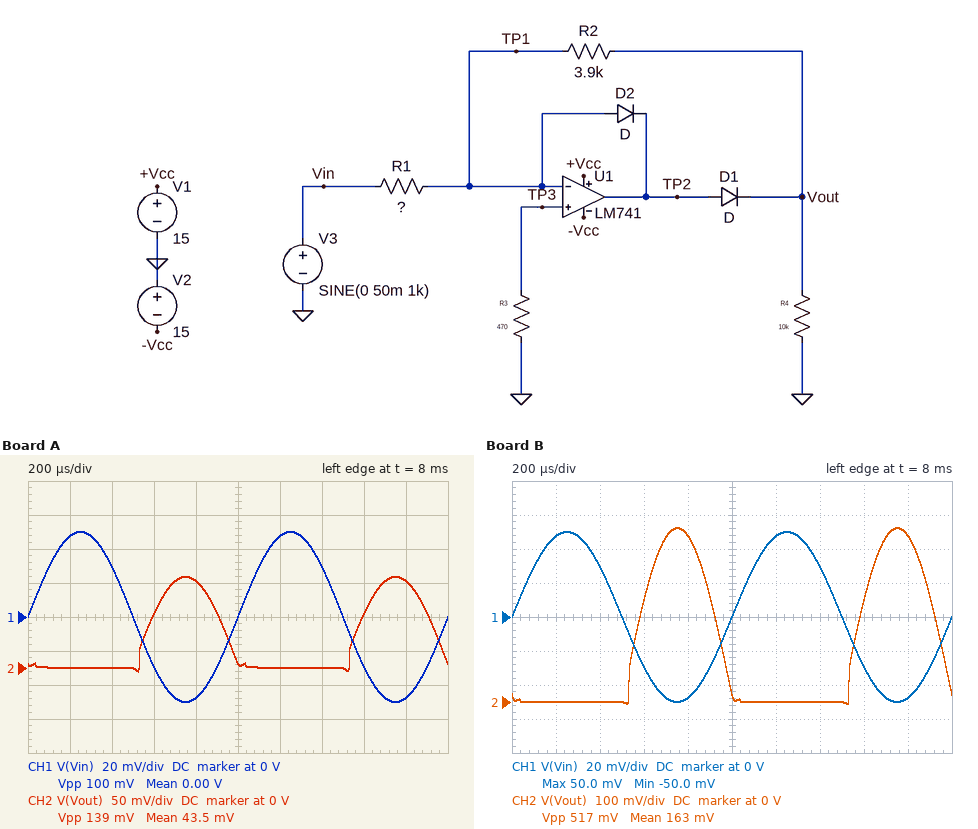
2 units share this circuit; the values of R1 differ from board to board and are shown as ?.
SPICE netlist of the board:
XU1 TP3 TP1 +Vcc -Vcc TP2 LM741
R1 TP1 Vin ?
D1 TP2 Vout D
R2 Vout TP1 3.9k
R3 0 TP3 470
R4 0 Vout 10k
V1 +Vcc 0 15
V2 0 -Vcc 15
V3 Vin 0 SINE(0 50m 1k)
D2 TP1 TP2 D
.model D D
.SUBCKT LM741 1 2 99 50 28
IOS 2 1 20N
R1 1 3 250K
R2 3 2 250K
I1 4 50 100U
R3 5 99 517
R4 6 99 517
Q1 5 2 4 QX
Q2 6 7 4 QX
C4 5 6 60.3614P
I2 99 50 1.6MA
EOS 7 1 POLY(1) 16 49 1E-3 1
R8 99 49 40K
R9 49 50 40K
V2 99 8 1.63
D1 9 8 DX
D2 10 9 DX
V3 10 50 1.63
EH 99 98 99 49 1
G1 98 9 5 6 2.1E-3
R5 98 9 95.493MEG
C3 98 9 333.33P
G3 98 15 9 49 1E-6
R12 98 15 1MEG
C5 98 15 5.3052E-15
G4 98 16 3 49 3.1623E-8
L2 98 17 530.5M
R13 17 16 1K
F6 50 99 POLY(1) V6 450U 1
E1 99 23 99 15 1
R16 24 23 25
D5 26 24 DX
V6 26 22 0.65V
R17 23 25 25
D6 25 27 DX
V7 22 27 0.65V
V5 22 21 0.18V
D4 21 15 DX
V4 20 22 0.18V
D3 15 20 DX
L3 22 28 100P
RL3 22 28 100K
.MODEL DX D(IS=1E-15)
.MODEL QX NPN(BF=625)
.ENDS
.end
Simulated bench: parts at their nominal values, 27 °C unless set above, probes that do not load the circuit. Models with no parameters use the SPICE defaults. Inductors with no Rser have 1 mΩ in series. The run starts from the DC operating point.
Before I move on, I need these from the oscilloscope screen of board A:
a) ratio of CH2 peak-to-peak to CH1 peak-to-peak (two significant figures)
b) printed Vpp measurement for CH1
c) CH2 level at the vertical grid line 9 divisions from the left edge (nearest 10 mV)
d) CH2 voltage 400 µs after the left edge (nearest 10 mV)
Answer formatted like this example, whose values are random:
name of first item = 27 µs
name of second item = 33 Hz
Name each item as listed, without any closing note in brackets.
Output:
ratio of CH2 peak-to-peak to CH1 peak-to-peak = 1.4
printed Vpp measurement for CH1 = 100 mV
CH2 level at the vertical grid line 9 divisions from the left edge = 130 mV
CH2 voltage 400 µs after the left edge = 0 V
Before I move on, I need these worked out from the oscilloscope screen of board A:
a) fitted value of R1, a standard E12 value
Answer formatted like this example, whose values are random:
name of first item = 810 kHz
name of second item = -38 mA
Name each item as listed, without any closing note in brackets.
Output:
fitted value of R1, a standard E12 value = 1.5 kΩ
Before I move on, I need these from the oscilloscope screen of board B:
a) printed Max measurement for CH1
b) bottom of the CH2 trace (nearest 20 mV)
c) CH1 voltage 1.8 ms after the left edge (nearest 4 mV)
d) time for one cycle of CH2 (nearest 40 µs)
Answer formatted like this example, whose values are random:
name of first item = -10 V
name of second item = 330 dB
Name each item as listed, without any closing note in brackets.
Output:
printed Max measurement for CH1 = 50.0 mV
bottom of the CH2 trace = 0 V
CH1 voltage 1.8 ms after the left edge = -48 mV
time for one cycle of CH2 = 1.00 ms
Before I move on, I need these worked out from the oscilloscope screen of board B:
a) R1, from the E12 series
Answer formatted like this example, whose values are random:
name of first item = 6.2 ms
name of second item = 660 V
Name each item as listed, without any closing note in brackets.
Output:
R1, from the E12 series = 390 Ω
